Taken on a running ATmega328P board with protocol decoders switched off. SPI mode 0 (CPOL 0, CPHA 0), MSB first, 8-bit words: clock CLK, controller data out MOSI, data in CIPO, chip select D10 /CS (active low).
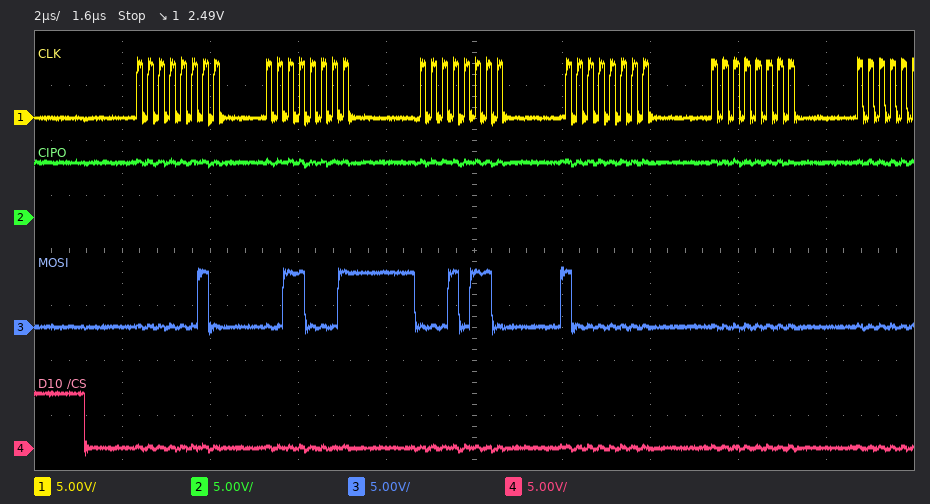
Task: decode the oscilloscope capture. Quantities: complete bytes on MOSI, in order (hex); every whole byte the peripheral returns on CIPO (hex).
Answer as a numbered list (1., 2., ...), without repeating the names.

1. 02 31 16 80 00
2. FF FF FF FF FF
